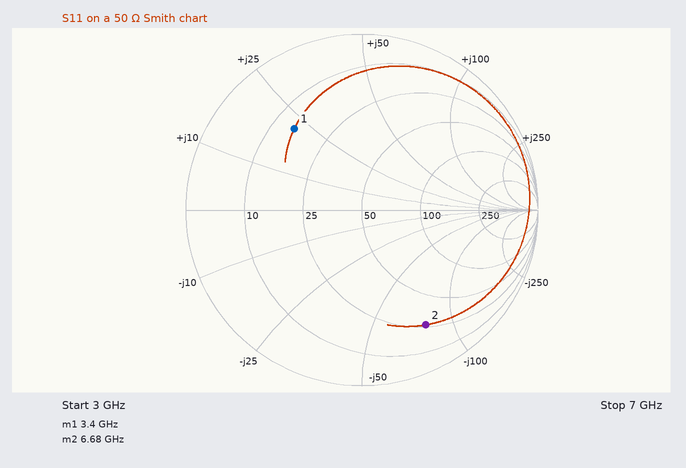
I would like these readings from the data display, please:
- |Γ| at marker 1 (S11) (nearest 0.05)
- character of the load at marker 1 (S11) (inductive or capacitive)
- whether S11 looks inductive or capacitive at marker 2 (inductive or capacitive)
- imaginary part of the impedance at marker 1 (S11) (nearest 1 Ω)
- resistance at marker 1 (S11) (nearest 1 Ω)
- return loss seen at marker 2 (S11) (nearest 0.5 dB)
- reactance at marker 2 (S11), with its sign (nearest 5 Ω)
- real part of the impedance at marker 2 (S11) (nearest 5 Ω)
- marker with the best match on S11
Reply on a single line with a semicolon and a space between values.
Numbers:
0.60; inductive; capacitive; +22 Ω; 15 Ω; 2.5 dB; -80 Ω; 25 Ω; marker 1
